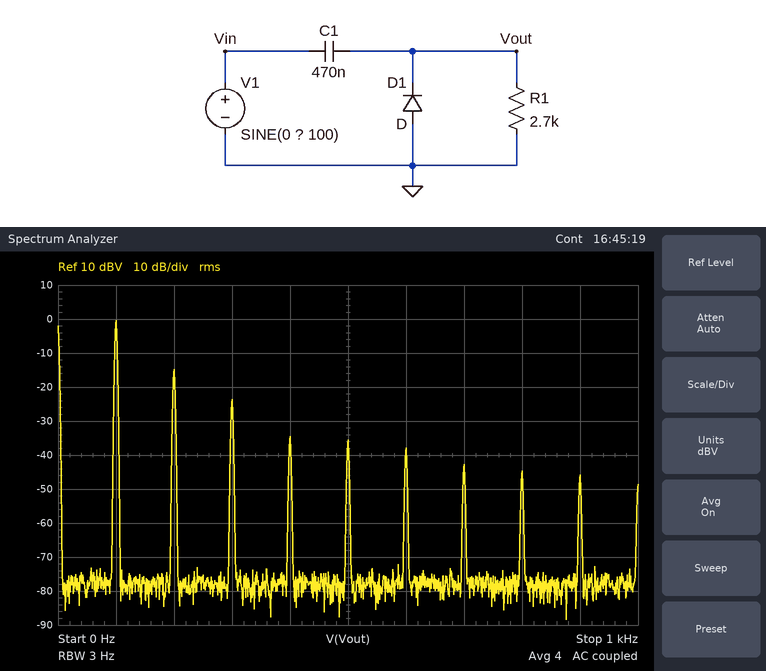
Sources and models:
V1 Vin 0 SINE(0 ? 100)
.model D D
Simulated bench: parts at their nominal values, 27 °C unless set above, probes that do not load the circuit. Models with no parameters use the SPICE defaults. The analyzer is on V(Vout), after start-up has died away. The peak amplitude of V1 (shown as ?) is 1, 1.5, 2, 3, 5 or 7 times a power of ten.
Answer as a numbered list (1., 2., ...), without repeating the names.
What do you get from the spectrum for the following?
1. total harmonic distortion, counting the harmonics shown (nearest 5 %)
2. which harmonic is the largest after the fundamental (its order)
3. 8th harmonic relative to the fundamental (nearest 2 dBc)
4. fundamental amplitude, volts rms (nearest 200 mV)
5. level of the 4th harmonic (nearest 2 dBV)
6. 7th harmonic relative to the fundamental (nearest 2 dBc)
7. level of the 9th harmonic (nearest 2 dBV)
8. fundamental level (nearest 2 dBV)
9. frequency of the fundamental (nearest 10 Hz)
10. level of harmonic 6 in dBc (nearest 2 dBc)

1. 20 %
2. 2
3. -44 dBc
4. 1.0 V
5. -34 dBV
6. -42 dBc
7. -46 dBV
8. 0 dBV
9. 100 Hz
10. -38 dBc
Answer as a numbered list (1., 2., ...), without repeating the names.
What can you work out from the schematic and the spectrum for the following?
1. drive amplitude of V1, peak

1. 3 V
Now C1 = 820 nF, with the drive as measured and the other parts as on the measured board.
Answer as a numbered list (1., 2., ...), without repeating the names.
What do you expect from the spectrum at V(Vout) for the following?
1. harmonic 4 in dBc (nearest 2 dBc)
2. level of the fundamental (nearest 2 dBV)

1. -32 dBc
2. 2 dBV
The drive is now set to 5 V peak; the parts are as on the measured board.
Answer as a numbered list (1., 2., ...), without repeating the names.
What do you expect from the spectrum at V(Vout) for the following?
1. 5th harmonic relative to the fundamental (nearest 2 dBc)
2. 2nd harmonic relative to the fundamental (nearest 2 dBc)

1. -32 dBc
2. -12 dBc
